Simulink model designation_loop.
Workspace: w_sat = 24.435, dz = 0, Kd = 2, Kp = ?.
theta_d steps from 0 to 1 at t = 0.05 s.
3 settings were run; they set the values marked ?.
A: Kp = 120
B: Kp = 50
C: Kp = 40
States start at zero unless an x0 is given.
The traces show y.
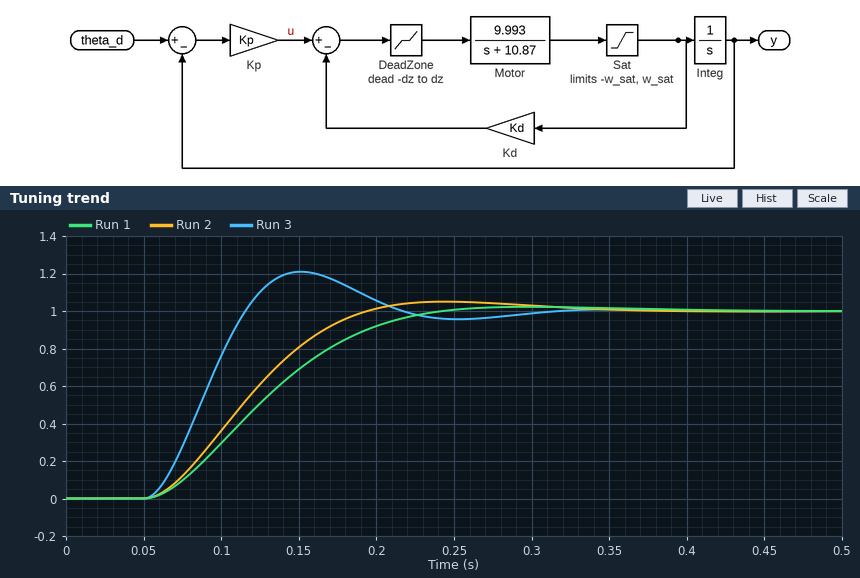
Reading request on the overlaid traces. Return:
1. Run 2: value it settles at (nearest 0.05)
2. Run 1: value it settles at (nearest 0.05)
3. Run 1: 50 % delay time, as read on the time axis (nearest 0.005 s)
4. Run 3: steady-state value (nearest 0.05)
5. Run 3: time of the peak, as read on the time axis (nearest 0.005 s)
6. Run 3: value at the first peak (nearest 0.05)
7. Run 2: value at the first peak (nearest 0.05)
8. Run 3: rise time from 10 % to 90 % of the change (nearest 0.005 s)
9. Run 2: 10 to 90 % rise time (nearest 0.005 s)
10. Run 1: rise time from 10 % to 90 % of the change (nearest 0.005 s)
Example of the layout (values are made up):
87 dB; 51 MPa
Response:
1.00; 1.00; 0.125 s; 1.00; 0.150 s; 1.20; 1.05; 0.045 s; 0.095 s; 0.120 s
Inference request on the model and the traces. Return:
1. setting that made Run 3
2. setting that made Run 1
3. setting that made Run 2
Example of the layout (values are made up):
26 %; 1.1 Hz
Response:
A; C; B
